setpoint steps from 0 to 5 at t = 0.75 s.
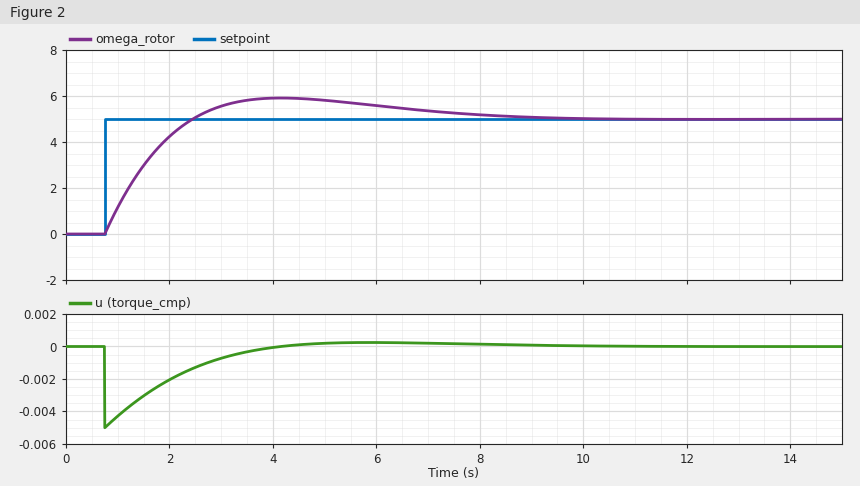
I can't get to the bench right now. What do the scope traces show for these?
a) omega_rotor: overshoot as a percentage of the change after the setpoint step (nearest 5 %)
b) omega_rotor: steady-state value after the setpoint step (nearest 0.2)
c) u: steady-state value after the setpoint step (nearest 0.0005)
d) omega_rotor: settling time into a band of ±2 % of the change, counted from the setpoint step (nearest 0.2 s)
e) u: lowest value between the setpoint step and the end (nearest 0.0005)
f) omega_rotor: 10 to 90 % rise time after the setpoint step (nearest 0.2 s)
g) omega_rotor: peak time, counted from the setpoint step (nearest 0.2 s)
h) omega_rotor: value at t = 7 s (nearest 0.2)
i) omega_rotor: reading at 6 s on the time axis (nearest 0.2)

20 %
5.0
0.0000
8.0 s
-0.0050
1.2 s
3.4 s
5.4
5.6
